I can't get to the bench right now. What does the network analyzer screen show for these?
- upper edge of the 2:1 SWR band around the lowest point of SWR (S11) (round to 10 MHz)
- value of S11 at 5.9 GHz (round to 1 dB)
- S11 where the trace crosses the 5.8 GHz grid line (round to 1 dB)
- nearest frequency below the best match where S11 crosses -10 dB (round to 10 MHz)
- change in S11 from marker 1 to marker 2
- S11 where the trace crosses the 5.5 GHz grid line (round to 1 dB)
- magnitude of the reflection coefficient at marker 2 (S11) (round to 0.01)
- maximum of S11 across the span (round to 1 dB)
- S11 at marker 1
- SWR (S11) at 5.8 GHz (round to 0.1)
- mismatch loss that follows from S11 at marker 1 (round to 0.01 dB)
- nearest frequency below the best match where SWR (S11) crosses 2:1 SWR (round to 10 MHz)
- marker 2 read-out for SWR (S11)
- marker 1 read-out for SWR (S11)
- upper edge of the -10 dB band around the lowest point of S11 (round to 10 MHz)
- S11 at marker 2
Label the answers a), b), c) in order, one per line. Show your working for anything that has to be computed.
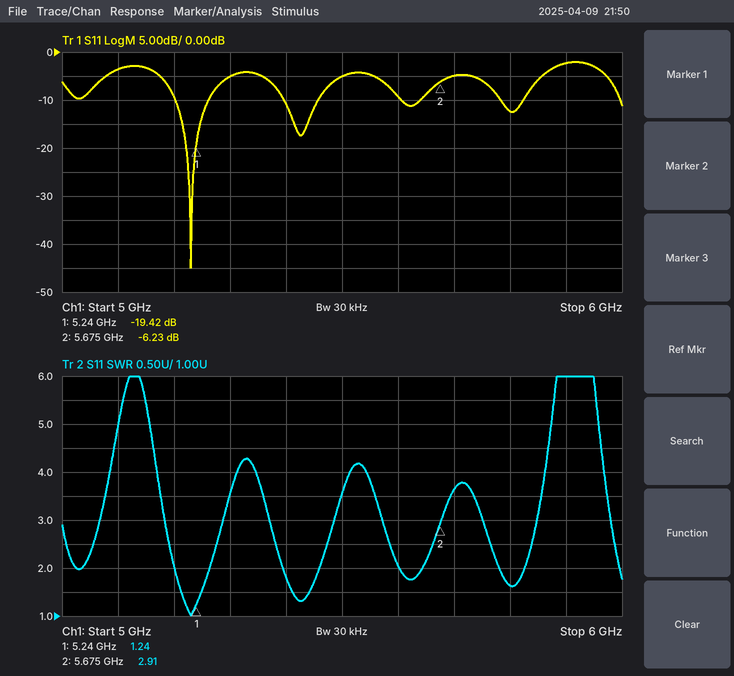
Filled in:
a) 5.26 GHz
b) -2 dB
c) -12 dB
d) 5.20 GHz
e) -6.23 − (-19.42) = 13.19 dB
f) -5 dB
g) 10^(-6.23/20) ≈ 0.49
h) -2 dB
i) -19.42 dB
j) 1.6
k) −10 log10(1 − 10^(-19.42/10)) ≈ 0.05 dB
l) 5.20 GHz
m) 2.91
n) 1.24
o) 5.26 GHz
p) -6.23 dB
